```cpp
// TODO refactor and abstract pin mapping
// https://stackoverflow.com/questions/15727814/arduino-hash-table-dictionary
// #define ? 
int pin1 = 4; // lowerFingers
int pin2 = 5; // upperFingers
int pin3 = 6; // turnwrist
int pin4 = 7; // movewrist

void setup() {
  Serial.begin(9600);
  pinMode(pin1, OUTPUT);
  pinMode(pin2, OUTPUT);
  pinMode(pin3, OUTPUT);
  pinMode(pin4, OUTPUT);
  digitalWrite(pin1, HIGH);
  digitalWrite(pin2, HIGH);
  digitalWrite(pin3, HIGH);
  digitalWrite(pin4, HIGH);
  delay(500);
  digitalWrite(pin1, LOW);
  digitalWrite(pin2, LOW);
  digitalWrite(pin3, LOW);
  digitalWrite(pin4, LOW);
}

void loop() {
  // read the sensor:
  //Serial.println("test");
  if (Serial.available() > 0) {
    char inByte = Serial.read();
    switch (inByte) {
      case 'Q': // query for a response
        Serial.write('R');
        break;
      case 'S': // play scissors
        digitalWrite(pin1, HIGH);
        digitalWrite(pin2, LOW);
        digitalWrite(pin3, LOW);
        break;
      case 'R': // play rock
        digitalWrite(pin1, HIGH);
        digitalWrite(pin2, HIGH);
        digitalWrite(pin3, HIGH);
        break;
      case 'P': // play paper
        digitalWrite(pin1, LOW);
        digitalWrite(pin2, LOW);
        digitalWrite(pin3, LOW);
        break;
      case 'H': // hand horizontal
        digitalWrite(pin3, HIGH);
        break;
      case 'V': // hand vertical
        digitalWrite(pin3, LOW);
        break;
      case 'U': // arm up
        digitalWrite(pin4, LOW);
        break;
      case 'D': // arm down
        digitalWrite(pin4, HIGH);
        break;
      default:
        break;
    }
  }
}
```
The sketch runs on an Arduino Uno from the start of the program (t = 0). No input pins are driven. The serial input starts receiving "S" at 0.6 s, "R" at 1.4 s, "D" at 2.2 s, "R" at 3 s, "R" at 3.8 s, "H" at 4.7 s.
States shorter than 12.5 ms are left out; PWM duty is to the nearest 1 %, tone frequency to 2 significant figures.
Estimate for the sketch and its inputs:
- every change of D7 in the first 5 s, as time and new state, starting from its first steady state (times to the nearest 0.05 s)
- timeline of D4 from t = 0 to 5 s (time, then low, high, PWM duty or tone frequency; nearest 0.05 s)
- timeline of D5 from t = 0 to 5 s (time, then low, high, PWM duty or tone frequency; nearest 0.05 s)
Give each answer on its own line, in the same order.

0 s high; 0.5 s low; 2.2 s high
0 s high; 0.5 s low; 0.6 s high
0 s high; 0.5 s low; 1.4 s high
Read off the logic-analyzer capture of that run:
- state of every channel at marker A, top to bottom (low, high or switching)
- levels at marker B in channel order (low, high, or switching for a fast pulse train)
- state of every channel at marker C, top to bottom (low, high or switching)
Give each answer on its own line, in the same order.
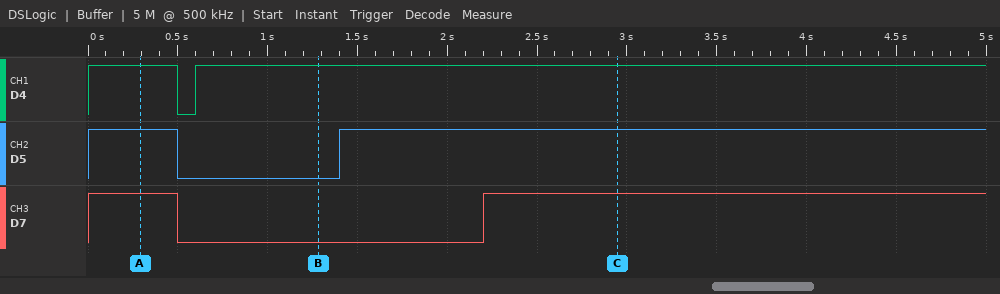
D4 high, D5 high, D7 high
D4 high, D5 low, D7 low
D4 high, D5 high, D7 high
